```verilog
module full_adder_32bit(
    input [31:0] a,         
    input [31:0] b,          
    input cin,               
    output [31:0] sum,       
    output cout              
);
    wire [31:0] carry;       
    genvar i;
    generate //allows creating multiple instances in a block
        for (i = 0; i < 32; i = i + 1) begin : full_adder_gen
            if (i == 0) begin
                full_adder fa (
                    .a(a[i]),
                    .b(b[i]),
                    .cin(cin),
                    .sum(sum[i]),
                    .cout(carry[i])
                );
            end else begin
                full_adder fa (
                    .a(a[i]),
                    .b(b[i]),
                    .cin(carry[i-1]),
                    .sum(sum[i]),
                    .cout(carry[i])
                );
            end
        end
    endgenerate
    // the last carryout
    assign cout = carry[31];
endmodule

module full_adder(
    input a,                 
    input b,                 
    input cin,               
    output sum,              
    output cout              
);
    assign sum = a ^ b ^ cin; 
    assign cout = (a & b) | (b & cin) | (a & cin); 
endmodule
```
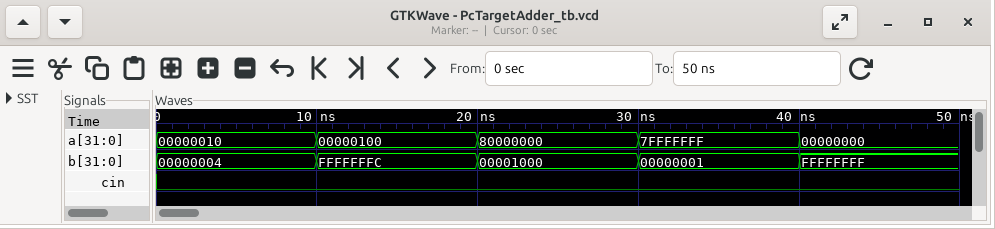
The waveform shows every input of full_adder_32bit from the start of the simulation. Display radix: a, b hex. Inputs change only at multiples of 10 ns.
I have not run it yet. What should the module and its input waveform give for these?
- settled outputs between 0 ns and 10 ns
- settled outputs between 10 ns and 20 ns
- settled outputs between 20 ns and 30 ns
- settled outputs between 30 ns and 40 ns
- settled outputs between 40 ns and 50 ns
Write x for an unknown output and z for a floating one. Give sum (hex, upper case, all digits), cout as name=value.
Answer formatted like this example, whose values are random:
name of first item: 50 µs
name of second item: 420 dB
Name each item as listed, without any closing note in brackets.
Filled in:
settled outputs between 0 ns and 10 ns: sum=00000014, cout=0
settled outputs between 10 ns and 20 ns: sum=000000FC, cout=1
settled outputs between 20 ns and 30 ns: sum=80001000, cout=0
settled outputs between 30 ns and 40 ns: sum=80000000, cout=0
settled outputs between 40 ns and 50 ns: sum=FFFFFFFF, cout=0
